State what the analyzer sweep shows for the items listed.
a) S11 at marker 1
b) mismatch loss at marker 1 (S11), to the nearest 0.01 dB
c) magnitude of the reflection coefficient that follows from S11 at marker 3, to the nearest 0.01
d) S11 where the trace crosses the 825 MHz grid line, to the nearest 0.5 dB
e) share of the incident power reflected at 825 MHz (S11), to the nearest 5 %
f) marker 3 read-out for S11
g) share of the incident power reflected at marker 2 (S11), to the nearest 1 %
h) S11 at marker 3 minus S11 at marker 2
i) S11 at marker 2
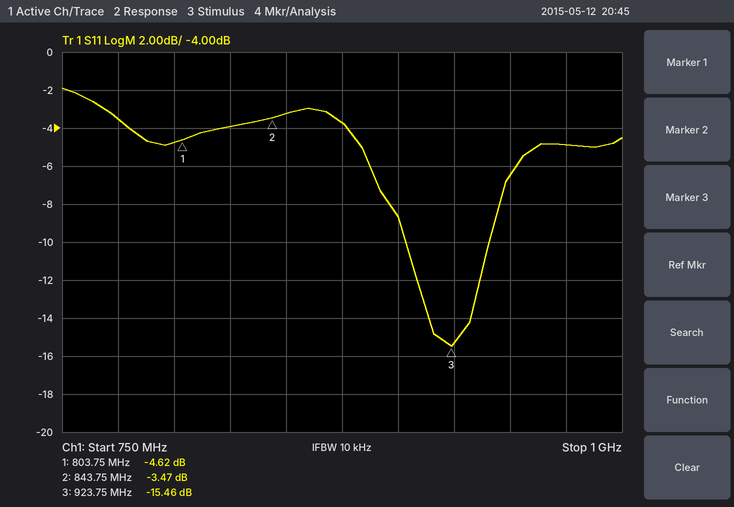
-4.62 dB
1.84 dB
0.17
-4.0 dB
40 %
-15.46 dB
45 %
-11.99 dB
-3.47 dB
